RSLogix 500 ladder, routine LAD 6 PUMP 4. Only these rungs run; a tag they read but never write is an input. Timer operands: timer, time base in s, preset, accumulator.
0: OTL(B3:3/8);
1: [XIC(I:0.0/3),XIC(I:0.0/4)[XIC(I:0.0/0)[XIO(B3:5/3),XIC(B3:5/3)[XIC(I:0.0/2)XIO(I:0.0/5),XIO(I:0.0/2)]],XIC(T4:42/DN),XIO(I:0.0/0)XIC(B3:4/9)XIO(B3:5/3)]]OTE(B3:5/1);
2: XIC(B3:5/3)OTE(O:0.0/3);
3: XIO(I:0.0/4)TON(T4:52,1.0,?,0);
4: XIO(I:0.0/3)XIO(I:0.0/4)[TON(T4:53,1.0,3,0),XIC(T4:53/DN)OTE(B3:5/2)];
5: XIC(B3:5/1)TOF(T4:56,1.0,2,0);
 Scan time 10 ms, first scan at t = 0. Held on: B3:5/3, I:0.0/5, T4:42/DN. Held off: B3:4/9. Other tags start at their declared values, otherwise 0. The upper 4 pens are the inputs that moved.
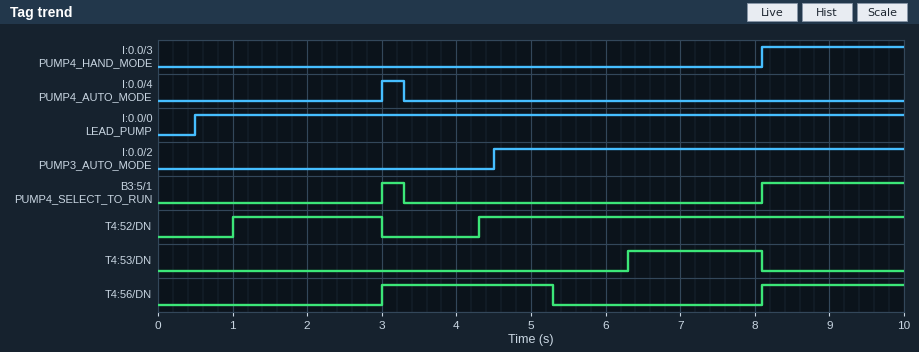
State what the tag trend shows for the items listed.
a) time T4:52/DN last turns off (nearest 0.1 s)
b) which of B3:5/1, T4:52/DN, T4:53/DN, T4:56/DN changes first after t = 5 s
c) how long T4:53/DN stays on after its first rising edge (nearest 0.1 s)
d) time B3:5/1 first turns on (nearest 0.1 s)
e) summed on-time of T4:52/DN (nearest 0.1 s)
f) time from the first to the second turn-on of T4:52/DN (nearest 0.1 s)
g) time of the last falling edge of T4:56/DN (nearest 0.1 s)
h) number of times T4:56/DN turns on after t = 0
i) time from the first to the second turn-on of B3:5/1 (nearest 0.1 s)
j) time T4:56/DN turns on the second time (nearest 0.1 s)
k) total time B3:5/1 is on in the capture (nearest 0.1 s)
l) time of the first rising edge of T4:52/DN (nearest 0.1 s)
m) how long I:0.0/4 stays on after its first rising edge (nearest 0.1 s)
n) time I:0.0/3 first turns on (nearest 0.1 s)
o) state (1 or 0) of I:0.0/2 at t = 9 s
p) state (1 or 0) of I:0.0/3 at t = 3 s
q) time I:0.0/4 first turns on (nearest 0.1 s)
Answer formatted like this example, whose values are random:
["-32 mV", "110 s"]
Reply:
["3.0 s", "T4:56/DN", "1.8 s", "3.0 s", "7.7 s", "3.3 s", "5.3 s", "2", "5.1 s", "8.1 s", "2.2 s", "1.0 s", "0.3 s", "8.1 s", "1", "0", "3.0 s"]
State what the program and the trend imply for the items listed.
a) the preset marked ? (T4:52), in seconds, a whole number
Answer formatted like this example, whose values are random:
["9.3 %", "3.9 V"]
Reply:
["1 s"]
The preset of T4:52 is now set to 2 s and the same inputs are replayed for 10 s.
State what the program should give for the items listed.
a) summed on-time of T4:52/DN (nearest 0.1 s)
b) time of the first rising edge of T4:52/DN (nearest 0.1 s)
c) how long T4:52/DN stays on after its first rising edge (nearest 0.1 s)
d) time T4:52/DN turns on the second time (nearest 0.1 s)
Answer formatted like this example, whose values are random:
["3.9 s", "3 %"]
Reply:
["5.7 s", "2.0 s", "1.0 s", "5.3 s"]
